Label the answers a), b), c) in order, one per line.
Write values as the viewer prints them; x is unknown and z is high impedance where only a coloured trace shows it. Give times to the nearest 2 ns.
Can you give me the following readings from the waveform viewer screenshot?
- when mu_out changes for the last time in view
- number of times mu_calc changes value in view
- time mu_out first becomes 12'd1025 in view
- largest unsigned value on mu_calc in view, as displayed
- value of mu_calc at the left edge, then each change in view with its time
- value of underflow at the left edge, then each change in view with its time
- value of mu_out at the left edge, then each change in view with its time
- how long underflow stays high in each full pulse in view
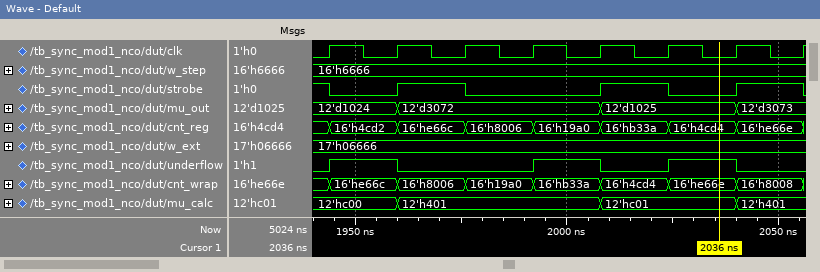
a) 2040 ns
b) 3
c) 2008 ns
d) 12'hc01
e) 12'hc00, 12'h401 at 1960 ns, 12'hc01 at 2008 ns, 12'h401 at 2040 ns
f) 0, 1 at 1944 ns, 0 at 1960 ns, 1 at 1992 ns, 0 at 2008 ns, 1 at 2024 ns, 0 at 2040 ns
g) 12'd1024, 12'd3072 at 1960 ns, 12'd1025 at 2008 ns, 12'd3073 at 2040 ns
h) 16 ns, 16 ns, 16 ns
